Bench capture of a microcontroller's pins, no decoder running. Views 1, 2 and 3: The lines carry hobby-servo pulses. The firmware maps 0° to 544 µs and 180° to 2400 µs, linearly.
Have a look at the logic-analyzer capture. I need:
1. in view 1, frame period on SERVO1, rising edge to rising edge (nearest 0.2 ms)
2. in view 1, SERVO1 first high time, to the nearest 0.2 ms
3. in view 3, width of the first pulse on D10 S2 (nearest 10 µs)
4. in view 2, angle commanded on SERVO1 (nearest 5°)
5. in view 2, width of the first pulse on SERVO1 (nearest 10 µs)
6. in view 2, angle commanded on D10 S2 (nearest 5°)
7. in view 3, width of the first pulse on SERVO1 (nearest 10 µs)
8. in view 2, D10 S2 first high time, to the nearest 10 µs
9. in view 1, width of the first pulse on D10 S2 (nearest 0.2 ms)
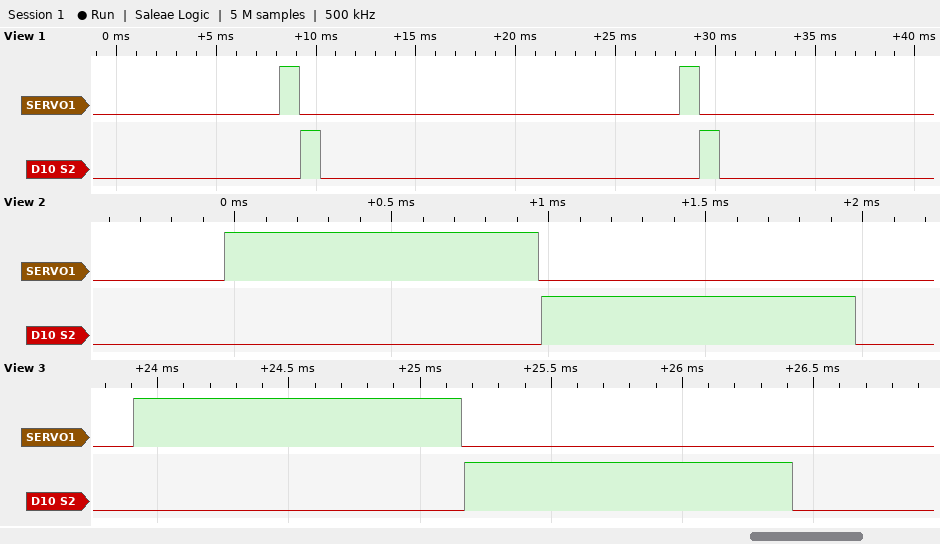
20.0 ms
1.0 ms
1250 µs
45°
1000 µs
45°
1250 µs
1000 µs
1.0 ms
